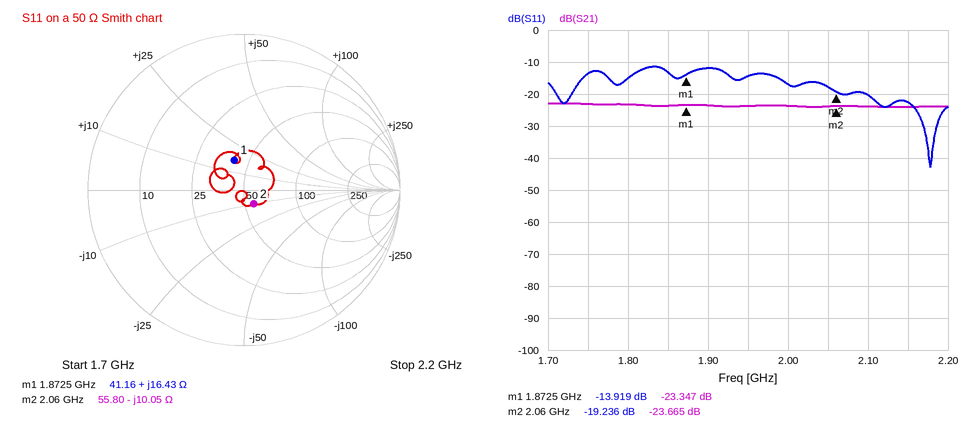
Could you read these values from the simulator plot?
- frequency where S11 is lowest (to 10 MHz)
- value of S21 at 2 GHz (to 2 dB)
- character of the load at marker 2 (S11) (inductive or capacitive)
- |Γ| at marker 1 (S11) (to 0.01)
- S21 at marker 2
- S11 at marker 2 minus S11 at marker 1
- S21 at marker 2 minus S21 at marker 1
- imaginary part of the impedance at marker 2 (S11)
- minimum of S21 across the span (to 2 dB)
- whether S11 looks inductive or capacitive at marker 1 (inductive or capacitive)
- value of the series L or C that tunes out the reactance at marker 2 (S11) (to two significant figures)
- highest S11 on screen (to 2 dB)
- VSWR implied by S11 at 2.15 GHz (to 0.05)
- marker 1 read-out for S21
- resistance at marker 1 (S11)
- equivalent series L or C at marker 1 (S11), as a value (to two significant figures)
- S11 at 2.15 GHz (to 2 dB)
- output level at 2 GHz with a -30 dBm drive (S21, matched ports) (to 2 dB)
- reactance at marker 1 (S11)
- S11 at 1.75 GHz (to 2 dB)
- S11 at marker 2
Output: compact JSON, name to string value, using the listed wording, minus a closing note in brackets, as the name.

{"frequency where S11 is lowest": "2.18 GHz", "value of S21 at 2 GHz": "-24 dB", "character of the load at marker 2 (S11)": "capacitive", "|Γ| at marker 1 (S11)": "0.20", "S21 at marker 2": "-23.665 dB", "S11 at marker 2 minus S11 at marker 1": "-5.317 dB", "S21 at marker 2 minus S21 at marker 1": "-0.318 dB", "imaginary part of the impedance at marker 2": "-10.05 Ω", "minimum of S21 across the span": "-24 dB", "whether S11 looks inductive or capacitive at marker 1": "inductive", "value of the series L or C that tunes out the reactance at marker 2 (S11)": "780 pH", "highest S11 on screen": "-12 dB", "VSWR implied by S11 at 2.15 GHz": "1.15", "marker 1 read-out for S21": "-23.347 dB", "resistance at marker 1": "41.16 Ω", "equivalent series L or C at marker 1 (S11), as a value": "1.4 nH", "S11 at 2.15 GHz": "-22 dB", "output level at 2 GHz with a -30 dBm drive (S21, matched ports)": "-54 dBm", "reactance at marker 1": "+16.43 Ω", "S11 at 1.75 GHz": "-14 dB", "S11 at marker 2": "-19.236 dB"}
